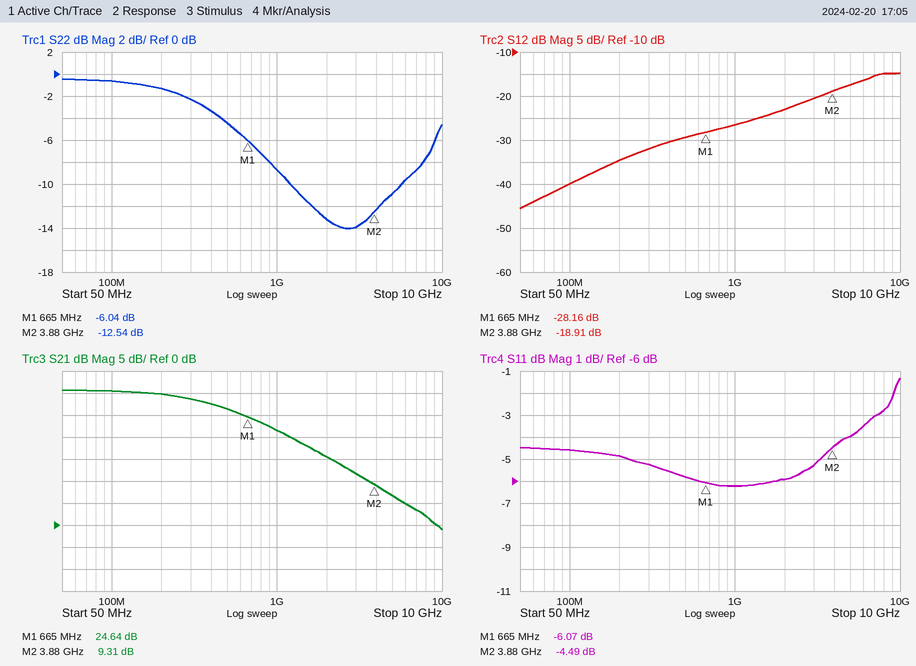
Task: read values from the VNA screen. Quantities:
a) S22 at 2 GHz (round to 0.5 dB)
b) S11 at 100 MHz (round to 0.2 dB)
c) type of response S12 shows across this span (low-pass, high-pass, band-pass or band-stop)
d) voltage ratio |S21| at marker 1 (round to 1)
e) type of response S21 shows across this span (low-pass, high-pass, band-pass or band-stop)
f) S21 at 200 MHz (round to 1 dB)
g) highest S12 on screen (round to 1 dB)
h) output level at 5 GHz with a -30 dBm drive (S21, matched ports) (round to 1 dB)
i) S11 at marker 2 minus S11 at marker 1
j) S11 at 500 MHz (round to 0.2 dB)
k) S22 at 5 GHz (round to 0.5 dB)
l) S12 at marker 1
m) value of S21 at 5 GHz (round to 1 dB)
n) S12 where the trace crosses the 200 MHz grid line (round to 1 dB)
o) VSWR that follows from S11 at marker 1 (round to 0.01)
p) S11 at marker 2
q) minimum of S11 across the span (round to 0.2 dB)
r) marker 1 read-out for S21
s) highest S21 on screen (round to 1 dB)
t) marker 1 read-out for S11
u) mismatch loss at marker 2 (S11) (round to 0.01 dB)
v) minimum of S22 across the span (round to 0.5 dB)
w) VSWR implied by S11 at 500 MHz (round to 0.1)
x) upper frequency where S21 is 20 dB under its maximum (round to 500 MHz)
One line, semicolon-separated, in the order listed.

-13.0 dB; -4.6 dB; high-pass; 17; low-pass; 30 dB; -15 dB; -23 dBm; 1.58 dB; -5.8 dB; -11.0 dB; -28.16 dB; 7 dB; -35 dB; 2.98; -4.49 dB; -6.2 dB; 24.64 dB; 31 dB; -6.07 dB; 1.91 dB; -14.0 dB; 3.1; 3.5 GHz
